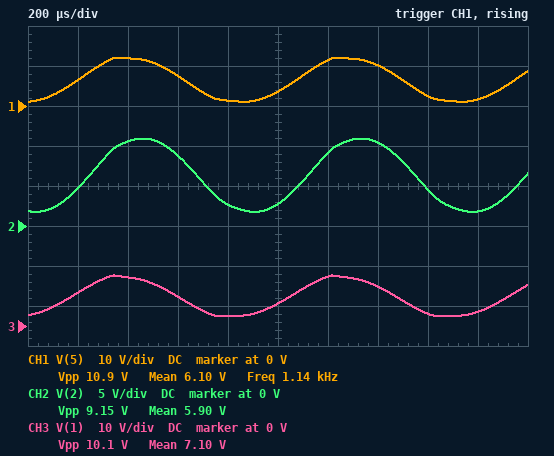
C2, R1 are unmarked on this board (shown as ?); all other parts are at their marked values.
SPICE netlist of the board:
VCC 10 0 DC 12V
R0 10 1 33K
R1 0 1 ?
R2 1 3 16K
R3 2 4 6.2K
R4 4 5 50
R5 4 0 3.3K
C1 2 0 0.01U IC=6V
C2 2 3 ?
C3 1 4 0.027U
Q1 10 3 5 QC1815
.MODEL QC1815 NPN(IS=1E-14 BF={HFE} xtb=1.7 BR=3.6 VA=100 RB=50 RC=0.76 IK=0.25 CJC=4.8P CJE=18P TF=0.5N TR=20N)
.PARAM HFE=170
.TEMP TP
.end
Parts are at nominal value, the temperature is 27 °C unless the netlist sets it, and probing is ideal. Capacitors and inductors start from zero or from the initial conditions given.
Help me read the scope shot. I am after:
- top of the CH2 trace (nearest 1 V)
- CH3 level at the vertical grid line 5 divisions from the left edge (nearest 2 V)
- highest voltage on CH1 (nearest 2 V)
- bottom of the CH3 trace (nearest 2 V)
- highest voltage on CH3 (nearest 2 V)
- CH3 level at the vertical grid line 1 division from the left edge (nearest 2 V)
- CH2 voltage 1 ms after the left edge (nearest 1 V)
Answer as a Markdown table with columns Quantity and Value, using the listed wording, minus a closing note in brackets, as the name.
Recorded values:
| Quantity | Value |
|---|---|
| top of the CH2 trace | 11 V |
| CH3 level at the vertical grid line 5 divisions from the left edge | 6 V |
| highest voltage on CH1 | 12 V |
| bottom of the CH3 trace | 2 V |
| highest voltage on CH3 | 12 V |
| CH3 level at the vertical grid line 1 division from the left edge | 8 V |
| CH2 voltage 1 ms after the left edge | 3 V |
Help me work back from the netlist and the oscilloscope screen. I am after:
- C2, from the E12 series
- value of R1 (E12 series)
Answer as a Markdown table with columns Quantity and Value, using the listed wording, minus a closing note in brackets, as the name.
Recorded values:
| Quantity | Value |
|---|---|
| C2, from the E12 series | 5.6 nF |
| value of R1 | 56 kΩ |
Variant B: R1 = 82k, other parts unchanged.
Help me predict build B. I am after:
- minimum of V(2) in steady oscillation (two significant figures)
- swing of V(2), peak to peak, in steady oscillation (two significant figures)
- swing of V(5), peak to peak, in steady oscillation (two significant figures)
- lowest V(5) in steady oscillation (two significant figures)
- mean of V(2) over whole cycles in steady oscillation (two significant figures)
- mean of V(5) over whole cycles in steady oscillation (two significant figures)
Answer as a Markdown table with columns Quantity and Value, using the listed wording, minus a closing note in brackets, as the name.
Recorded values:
| Quantity | Value |
|---|---|
| minimum of V(2) in steady oscillation | 2.7 V |
| swing of V(2), peak to peak, in steady oscillation | 8.4 V |
| swing of V(5), peak to peak, in steady oscillation | 9.9 V |
| lowest V(5) in steady oscillation | 2.0 V |
| mean of V(2) over whole cycles in steady oscillation | 7.1 V |
| mean of V(5) over whole cycles in steady oscillation | 7.2 V |
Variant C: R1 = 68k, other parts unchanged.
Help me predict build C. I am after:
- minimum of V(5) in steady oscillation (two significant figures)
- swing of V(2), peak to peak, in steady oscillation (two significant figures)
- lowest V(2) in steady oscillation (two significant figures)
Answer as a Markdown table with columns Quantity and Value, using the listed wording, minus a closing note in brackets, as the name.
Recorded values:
| Quantity | Value |
|---|---|
| minimum of V(5) in steady oscillation | 1.3 V |
| swing of V(2), peak to peak, in steady oscillation | 9.0 V |
| lowest V(2) in steady oscillation | 2.0 V |
